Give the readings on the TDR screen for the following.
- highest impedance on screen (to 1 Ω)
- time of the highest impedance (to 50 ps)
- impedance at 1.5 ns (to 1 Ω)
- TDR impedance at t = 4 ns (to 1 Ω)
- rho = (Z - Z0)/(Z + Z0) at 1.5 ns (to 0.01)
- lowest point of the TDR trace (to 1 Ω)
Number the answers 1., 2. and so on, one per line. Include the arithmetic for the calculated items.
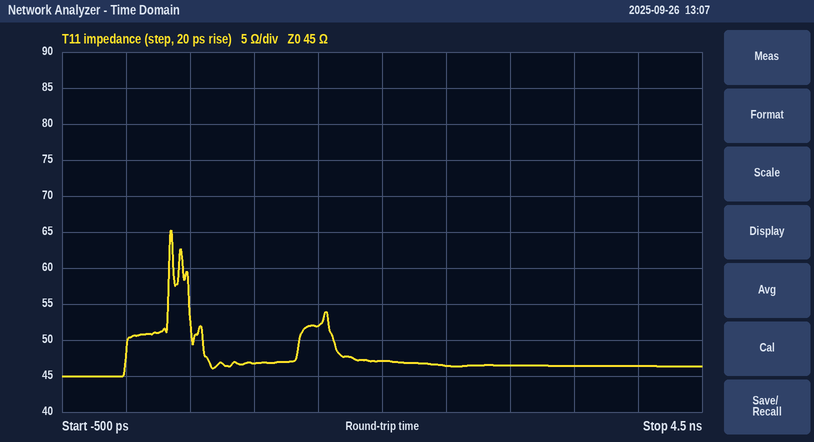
1. 65 Ω
2. 350 ps
3. 52 Ω
4. 46 Ω
5. (52 − 45)/(52 + 45) ≈ +0.07
6. 45 Ω
